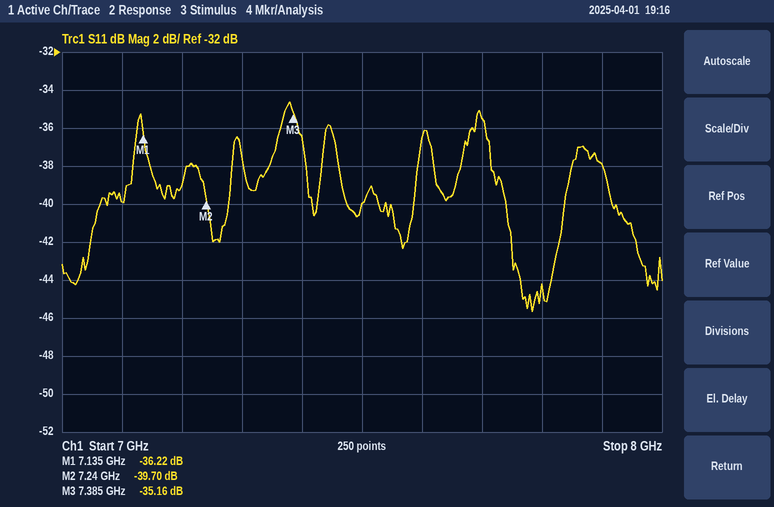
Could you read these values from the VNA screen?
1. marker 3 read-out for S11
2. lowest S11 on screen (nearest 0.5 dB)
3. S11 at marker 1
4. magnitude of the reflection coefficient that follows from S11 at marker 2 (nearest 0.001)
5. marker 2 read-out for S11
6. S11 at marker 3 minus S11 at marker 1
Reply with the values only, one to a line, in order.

-35.16 dB
-45.5 dB
-36.22 dB
0.010
-39.70 dB
1.06 dB
